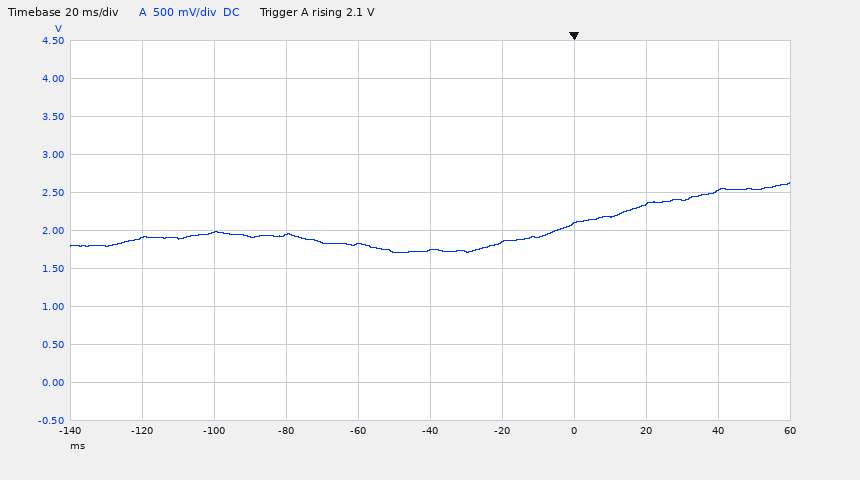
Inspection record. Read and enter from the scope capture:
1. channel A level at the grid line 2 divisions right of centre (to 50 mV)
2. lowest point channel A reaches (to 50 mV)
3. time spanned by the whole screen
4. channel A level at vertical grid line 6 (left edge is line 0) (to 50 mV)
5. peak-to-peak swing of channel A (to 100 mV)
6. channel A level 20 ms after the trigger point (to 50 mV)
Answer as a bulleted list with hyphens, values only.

- 2.10 V
- 1.70 V
- 200 ms
- 1.85 V
- 900 mV
- 2.35 V
